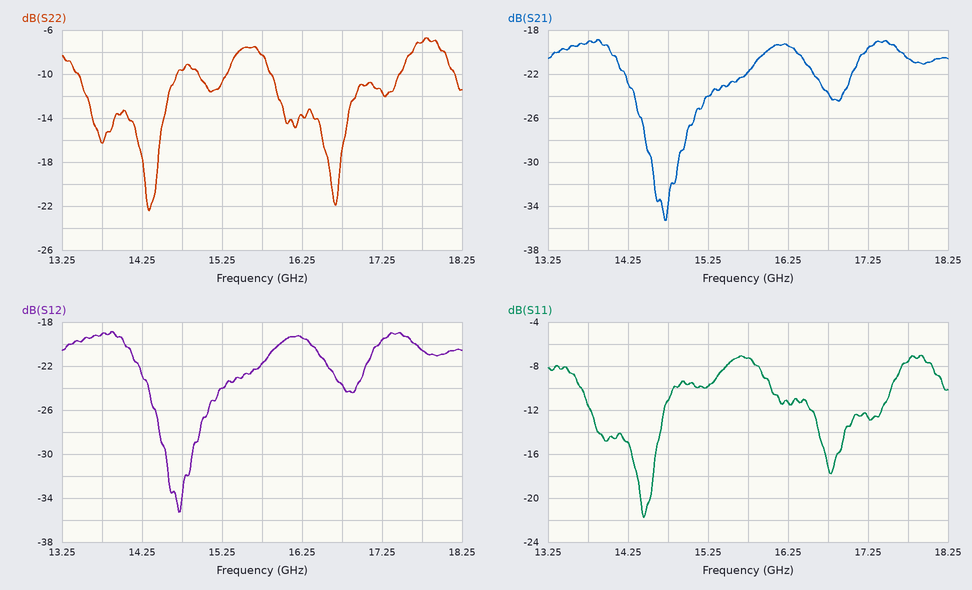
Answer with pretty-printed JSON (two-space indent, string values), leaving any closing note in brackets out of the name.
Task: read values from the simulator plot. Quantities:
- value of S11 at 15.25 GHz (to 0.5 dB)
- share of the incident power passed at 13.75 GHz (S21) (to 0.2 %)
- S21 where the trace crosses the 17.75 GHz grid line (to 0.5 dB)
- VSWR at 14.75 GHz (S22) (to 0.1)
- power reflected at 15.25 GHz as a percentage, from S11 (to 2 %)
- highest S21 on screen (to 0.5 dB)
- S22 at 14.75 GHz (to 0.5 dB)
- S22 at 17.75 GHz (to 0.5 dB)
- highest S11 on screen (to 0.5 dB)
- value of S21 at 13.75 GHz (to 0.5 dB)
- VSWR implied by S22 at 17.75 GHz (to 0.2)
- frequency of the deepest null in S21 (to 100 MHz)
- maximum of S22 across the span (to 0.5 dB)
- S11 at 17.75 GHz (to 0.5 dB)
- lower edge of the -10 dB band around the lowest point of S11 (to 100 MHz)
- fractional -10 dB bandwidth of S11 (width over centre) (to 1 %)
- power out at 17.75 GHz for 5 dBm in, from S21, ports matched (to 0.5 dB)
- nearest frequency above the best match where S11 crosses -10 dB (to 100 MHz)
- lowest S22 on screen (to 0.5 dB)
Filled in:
{
  "value of S11 at 15.25 GHz": "-10.0 dB",
  "share of the incident power passed at 13.75 GHz (S21)": "1.2 %",
  "S21 where the trace crosses the 17.75 GHz grid line": "-20.5 dB",
  "VSWR at 14.75 GHz (S22)": "2.0",
  "power reflected at 15.25 GHz as a percentage, from S11": "10 %",
  "highest S21 on screen": "-19.0 dB",
  "S22 at 14.75 GHz": "-9.5 dB",
  "S22 at 17.75 GHz": "-7.0 dB",
  "highest S11 on screen": "-7.0 dB",
  "value of S21 at 13.75 GHz": "-19.0 dB",
  "VSWR implied by S22 at 17.75 GHz": "2.6",
  "frequency of the deepest null in S21": "14.7 GHz",
  "maximum of S22 across the span": "-6.5 dB",
  "S11 at 17.75 GHz": "-7.5 dB",
  "lower edge of the -10 dB band around the lowest point of S11": "13.7 GHz",
  "fractional -10 dB bandwidth of S11 (width over centre)": "8 %",
  "power out at 17.75 GHz for 5 dBm in, from S21, ports matched": "-15.5 dBm",
  "nearest frequency above the best match where S11 crosses -10 dB": "14.8 GHz",
  "lowest S22 on screen": "-22.5 dB"
}
